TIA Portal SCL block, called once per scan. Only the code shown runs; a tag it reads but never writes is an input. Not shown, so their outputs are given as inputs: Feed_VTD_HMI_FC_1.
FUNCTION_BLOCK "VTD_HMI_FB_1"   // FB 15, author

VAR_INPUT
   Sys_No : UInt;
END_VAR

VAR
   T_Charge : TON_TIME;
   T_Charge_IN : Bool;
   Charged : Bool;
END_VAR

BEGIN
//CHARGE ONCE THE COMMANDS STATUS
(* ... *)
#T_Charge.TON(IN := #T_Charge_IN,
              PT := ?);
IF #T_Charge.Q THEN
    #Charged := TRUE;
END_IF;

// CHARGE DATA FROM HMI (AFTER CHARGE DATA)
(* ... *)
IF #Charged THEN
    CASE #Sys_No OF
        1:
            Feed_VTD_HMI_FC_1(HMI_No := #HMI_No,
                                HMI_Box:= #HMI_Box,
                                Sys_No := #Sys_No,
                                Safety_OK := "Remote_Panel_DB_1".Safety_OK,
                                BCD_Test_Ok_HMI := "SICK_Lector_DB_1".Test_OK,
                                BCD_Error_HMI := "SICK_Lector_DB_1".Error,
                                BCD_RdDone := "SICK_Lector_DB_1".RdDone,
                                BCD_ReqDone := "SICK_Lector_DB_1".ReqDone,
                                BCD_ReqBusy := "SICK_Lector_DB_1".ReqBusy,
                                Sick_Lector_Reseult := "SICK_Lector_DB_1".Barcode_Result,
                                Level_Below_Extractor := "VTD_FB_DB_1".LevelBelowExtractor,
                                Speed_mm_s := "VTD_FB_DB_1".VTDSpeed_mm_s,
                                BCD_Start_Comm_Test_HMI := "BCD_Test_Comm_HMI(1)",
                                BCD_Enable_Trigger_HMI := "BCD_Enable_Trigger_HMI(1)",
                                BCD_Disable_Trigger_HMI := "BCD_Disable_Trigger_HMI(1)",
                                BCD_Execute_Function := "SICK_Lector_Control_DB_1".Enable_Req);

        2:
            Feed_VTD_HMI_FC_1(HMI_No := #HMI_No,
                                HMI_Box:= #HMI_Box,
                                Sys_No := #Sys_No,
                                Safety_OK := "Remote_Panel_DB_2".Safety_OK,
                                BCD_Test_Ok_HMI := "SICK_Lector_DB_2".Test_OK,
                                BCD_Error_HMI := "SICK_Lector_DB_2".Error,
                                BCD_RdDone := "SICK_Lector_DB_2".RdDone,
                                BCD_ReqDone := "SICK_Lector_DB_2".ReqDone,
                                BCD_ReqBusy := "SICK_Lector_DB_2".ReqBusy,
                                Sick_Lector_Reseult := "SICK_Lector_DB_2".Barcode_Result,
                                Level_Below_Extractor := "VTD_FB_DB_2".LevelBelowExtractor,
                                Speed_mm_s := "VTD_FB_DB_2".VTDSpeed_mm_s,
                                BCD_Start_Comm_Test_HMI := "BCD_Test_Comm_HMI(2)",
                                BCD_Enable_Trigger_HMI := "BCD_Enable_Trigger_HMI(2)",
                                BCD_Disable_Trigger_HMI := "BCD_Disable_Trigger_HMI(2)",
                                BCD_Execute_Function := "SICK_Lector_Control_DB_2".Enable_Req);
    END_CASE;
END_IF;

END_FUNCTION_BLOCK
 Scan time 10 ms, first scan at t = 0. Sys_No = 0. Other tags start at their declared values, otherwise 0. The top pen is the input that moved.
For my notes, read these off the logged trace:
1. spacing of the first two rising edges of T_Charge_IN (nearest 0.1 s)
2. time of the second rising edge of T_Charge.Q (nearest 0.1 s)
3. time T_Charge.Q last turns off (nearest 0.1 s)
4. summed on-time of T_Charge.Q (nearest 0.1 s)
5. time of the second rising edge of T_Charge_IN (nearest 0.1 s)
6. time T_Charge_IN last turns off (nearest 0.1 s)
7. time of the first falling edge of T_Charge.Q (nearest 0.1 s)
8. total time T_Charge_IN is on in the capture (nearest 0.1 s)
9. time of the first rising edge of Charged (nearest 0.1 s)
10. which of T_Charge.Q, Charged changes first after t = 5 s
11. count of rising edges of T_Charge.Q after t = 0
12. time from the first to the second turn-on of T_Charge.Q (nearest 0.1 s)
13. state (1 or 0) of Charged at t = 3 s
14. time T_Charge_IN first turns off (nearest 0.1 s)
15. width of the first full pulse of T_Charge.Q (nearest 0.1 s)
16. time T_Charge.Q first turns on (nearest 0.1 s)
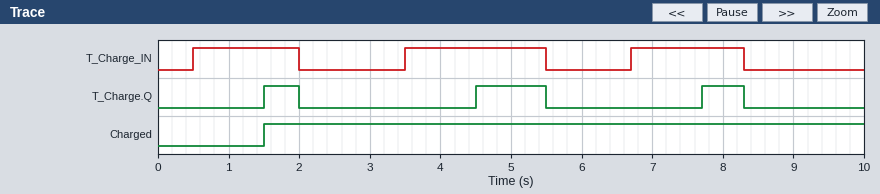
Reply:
3.0 s
4.5 s
8.3 s
2.1 s
3.5 s
8.3 s
2.0 s
5.1 s
1.5 s
T_Charge.Q
3
3.0 s
1
2.0 s
0.5 s
1.5 s
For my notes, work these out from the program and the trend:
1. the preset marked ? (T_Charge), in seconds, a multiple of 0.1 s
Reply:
1.0 s
